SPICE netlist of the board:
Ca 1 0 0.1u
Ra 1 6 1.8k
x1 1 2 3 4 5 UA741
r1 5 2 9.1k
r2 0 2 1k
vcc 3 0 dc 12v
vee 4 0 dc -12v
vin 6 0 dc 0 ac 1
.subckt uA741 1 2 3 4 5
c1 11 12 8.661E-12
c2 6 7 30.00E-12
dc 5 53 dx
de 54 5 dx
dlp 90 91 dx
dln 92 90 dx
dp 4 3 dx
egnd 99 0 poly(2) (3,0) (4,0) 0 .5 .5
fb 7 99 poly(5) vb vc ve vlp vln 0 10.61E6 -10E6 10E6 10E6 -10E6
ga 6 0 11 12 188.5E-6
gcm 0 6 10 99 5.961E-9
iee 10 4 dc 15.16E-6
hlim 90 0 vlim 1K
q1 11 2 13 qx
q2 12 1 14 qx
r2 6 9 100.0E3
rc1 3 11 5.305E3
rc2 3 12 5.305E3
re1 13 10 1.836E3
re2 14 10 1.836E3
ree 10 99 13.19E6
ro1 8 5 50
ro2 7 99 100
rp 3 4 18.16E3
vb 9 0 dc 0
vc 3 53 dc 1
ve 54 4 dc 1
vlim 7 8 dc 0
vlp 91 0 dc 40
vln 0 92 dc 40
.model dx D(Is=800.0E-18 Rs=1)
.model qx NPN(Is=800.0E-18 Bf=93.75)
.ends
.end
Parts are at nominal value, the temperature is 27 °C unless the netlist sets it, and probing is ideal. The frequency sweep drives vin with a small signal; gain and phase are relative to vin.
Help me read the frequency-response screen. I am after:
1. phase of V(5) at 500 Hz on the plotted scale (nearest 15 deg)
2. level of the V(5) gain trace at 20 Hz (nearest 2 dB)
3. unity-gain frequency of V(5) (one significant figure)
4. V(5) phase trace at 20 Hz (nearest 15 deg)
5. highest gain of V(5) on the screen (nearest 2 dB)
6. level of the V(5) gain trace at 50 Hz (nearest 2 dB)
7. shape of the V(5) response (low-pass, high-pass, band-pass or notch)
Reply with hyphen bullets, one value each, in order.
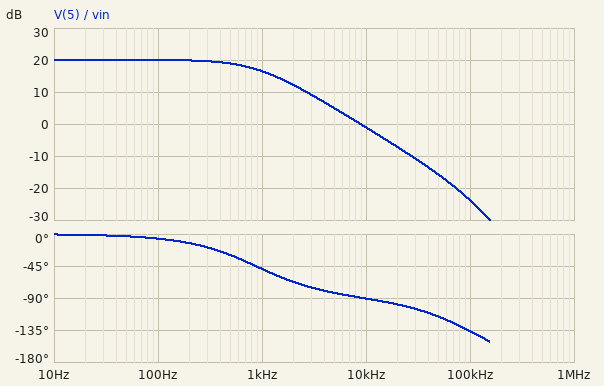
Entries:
- -30 deg
- 20 dB
- 9 kHz
- 0 deg
- 20 dB
- 20 dB
- low-pass
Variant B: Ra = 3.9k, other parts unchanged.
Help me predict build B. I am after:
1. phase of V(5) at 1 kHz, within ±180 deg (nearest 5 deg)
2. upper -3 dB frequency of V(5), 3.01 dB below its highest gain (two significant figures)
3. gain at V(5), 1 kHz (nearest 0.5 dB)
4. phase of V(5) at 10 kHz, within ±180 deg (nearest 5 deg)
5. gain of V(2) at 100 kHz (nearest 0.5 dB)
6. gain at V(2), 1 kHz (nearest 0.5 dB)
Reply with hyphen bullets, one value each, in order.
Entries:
- -70 deg
- 410 Hz
- 11.5 dB
- -95 deg
- -50.5 dB
- -8.5 dB
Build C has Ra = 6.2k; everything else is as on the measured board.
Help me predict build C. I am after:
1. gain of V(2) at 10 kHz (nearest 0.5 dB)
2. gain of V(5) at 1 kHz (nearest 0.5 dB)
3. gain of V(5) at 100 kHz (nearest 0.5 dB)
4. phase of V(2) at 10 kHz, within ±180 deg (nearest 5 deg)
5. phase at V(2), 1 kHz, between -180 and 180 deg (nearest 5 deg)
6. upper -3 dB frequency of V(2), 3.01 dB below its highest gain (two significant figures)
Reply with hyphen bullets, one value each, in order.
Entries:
- -32.0 dB
- 8.0 dB
- -34.5 dB
- -95 deg
- -75 deg
- 260 Hz
